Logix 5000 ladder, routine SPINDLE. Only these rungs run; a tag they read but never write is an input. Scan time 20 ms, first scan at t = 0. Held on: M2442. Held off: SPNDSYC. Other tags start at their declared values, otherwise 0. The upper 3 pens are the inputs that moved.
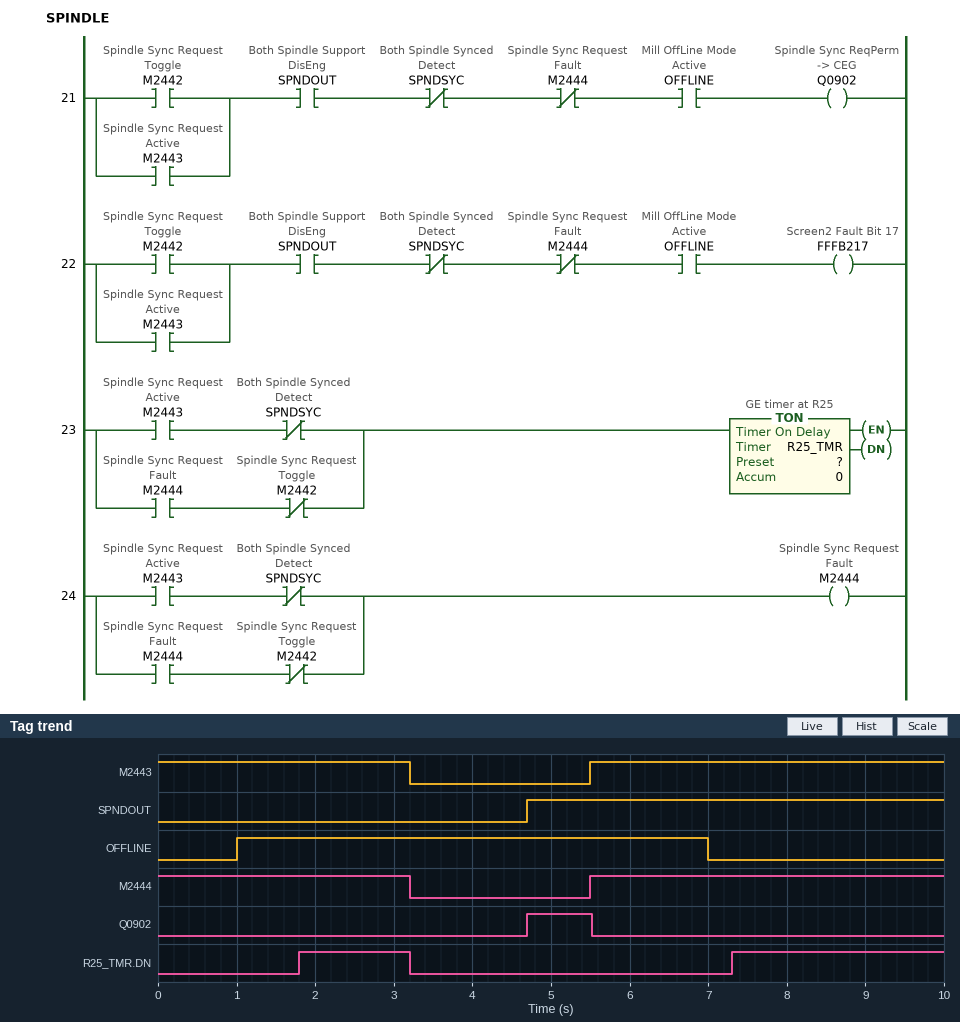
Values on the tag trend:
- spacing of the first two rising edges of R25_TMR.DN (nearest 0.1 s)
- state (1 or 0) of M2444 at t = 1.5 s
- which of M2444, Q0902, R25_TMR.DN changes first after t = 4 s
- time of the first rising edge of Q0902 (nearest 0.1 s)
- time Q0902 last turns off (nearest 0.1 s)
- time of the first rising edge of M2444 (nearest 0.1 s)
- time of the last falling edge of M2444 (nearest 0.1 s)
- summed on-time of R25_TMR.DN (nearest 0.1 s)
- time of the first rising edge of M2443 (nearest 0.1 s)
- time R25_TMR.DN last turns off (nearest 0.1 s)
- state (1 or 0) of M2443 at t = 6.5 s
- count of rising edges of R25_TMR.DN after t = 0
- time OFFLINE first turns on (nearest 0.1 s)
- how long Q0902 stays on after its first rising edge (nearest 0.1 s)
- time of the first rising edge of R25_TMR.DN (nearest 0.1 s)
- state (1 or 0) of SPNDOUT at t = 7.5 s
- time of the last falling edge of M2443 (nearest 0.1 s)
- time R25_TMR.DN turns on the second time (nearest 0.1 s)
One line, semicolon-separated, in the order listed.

5.5 s; 1; Q0902; 4.7 s; 5.5 s; 5.5 s; 3.2 s; 4.1 s; 5.5 s; 3.2 s; 1; 2; 1.0 s; 0.8 s; 1.8 s; 1; 3.2 s; 7.3 s
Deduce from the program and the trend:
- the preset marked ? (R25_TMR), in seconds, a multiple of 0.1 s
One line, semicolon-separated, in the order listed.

1.8 s
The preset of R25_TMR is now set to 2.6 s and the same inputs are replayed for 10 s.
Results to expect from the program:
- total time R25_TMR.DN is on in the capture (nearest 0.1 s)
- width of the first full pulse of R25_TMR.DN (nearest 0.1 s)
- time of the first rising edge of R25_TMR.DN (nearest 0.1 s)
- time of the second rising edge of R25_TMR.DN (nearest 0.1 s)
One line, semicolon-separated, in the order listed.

2.5 s; 0.6 s; 2.6 s; 8.1 s
